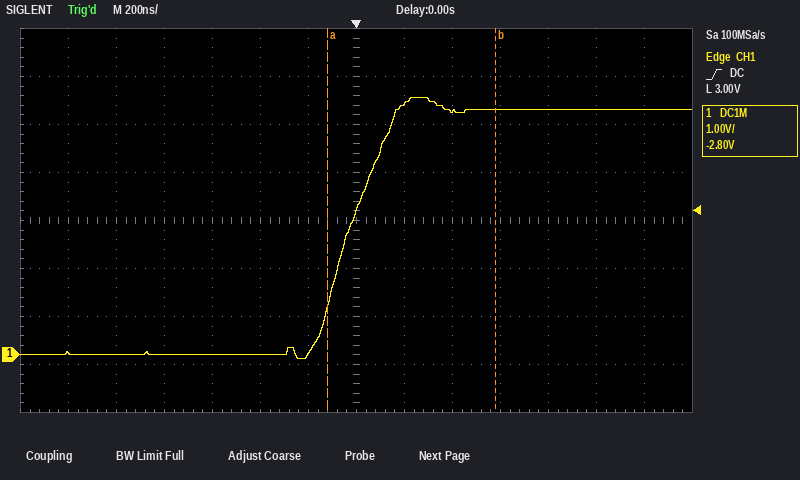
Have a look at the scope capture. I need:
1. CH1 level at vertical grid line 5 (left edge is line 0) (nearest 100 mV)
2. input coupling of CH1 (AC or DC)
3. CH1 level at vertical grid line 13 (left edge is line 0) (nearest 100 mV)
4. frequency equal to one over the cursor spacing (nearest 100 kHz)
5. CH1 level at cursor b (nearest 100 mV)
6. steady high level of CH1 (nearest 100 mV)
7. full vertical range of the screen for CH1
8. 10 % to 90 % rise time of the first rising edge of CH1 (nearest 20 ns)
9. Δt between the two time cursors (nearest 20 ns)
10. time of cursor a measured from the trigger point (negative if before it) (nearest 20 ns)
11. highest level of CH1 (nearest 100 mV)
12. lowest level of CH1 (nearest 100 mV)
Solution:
0.0 V
DC
5.1 V
1.4 MHz
5.1 V
5.1 V
8 V
280 ns
700 ns
-120 ns
5.4 V
-100 mV
